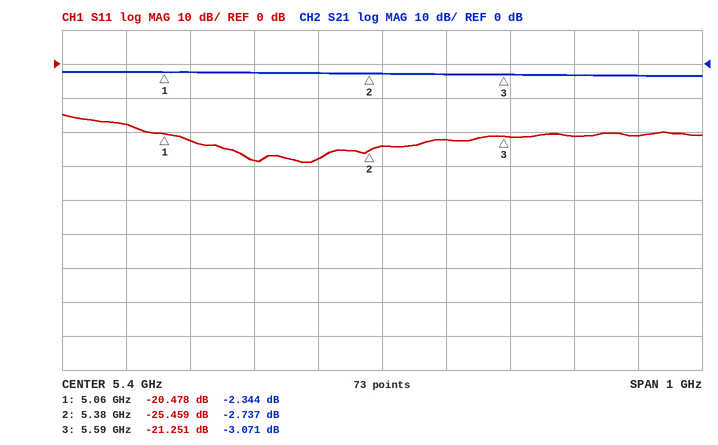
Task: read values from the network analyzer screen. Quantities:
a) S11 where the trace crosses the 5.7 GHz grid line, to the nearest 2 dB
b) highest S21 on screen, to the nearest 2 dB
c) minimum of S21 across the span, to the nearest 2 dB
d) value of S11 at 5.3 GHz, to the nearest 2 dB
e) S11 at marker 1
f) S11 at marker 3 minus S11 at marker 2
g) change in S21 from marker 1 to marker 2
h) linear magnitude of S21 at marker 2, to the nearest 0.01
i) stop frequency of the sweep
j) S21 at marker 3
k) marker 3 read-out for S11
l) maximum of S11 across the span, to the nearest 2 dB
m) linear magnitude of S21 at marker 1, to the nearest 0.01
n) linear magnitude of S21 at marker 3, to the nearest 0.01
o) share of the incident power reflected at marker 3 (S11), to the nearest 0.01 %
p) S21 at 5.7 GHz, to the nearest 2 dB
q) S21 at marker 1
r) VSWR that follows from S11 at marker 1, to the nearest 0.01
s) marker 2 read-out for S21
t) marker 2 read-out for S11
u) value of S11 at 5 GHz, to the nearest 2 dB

-22 dB
-2 dB
-4 dB
-28 dB
-20.478 dB
4.208 dB
-0.393 dB
0.73
5.9 GHz
-3.071 dB
-21.251 dB
-14 dB
0.76
0.70
0.75 %
-4 dB
-2.344 dB
1.21
-2.737 dB
-25.459 dB
-18 dB
